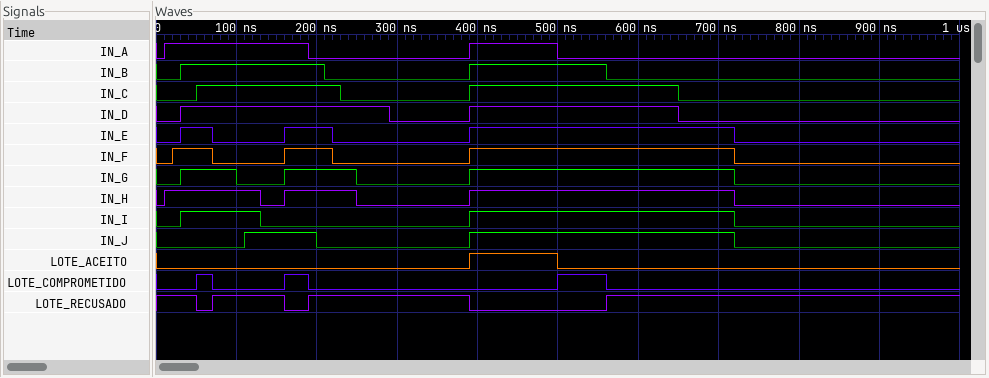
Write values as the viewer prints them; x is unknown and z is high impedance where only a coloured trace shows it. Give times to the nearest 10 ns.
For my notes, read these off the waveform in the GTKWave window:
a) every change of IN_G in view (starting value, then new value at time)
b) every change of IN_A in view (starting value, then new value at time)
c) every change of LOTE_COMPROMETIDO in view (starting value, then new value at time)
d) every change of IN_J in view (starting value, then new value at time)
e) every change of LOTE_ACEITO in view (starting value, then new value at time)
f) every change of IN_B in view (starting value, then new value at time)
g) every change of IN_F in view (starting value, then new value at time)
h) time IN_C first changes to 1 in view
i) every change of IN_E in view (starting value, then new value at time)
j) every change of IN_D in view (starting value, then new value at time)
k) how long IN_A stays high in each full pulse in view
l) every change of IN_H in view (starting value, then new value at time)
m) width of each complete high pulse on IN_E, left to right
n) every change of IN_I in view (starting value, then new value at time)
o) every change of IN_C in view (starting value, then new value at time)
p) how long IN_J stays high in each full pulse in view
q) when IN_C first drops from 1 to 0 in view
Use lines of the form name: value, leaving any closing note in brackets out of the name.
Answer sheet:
every change of IN_G in view: 0, 1 at 30 ns, 0 at 100 ns, 1 at 160 ns, 0 at 250 ns, 1 at 390 ns, 0 at 720 ns
every change of IN_A in view: 0, 1 at 10 ns, 0 at 190 ns, 1 at 390 ns, 0 at 500 ns
every change of LOTE_COMPROMETIDO in view: 0, 1 at 50 ns, 0 at 70 ns, 1 at 160 ns, 0 at 190 ns, 1 at 500 ns, 0 at 560 ns
every change of IN_J in view: 0, 1 at 110 ns, 0 at 200 ns, 1 at 390 ns, 0 at 720 ns
every change of LOTE_ACEITO in view: 0, 1 at 390 ns, 0 at 500 ns
every change of IN_B in view: 0, 1 at 30 ns, 0 at 210 ns, 1 at 390 ns, 0 at 560 ns
every change of IN_F in view: 0, 1 at 20 ns, 0 at 70 ns, 1 at 160 ns, 0 at 220 ns, 1 at 390 ns, 0 at 720 ns
time IN_C first changes to 1 in view: 50 ns
every change of IN_E in view: 0, 1 at 30 ns, 0 at 70 ns, 1 at 160 ns, 0 at 220 ns, 1 at 390 ns, 0 at 720 ns
every change of IN_D in view: 0, 1 at 30 ns, 0 at 290 ns, 1 at 390 ns, 0 at 650 ns
how long IN_A stays high in each full pulse in view: 180 ns, 110 ns
every change of IN_H in view: 0, 1 at 10 ns, 0 at 130 ns, 1 at 160 ns, 0 at 250 ns, 1 at 390 ns, 0 at 720 ns
width of each complete high pulse on IN_E, left to right: 40 ns, 60 ns, 330 ns
every change of IN_I in view: 0, 1 at 30 ns, 0 at 130 ns, 1 at 390 ns, 0 at 720 ns
every change of IN_C in view: 0, 1 at 50 ns, 0 at 230 ns, 1 at 390 ns, 0 at 650 ns
how long IN_J stays high in each full pulse in view: 90 ns, 330 ns
when IN_C first drops from 1 to 0 in view: 230 ns
